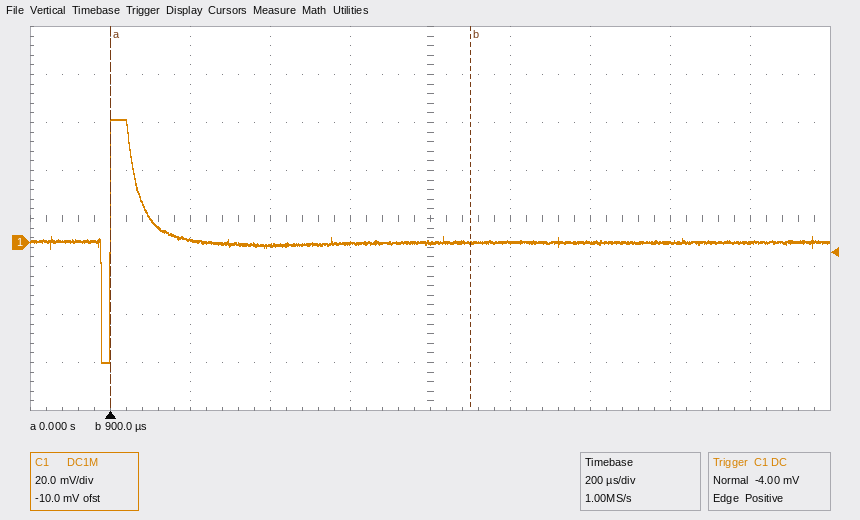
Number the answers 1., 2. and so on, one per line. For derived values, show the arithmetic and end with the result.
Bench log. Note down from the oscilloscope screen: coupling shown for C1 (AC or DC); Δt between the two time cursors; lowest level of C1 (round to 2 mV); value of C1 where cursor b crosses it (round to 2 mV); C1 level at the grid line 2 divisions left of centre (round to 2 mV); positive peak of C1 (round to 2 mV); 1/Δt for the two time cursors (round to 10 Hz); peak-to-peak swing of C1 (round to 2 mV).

1. DC
2. 900 µs − (0 s) = 900 µs
3. -50 mV
4. 0 mV
5. -2 mV
6. 52 mV
7. 1 / 900 µs ≈ 1.11 kHz
8. 52 mV − (-50 mV) = 102 mV
